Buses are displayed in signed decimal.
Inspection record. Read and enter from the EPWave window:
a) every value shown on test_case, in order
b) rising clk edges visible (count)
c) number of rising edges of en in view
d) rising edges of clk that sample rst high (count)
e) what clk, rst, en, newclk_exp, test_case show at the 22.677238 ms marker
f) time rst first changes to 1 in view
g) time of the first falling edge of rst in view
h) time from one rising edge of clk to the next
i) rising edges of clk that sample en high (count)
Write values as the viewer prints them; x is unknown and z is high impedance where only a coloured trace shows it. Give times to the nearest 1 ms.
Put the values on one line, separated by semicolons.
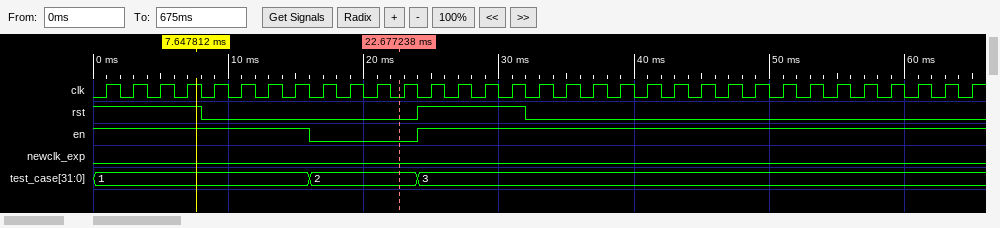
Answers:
1, 2, 3; 33; 1; 8; clk=0, rst=0, en=0, newclk_exp=0, test_case=2; 24 ms; 8 ms; 2 ms; 29
